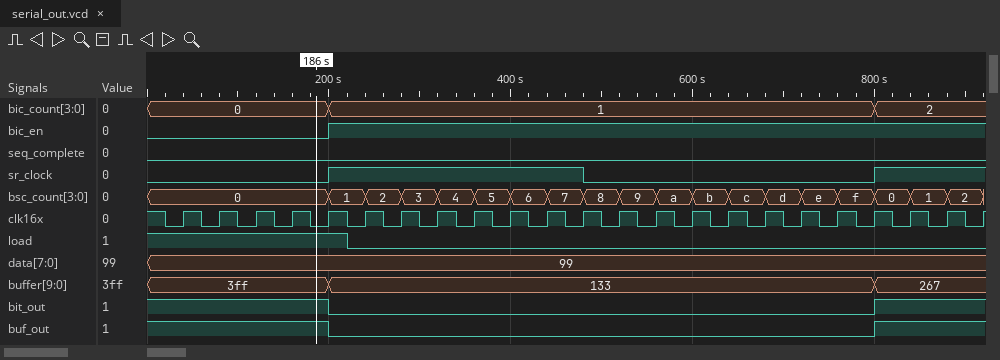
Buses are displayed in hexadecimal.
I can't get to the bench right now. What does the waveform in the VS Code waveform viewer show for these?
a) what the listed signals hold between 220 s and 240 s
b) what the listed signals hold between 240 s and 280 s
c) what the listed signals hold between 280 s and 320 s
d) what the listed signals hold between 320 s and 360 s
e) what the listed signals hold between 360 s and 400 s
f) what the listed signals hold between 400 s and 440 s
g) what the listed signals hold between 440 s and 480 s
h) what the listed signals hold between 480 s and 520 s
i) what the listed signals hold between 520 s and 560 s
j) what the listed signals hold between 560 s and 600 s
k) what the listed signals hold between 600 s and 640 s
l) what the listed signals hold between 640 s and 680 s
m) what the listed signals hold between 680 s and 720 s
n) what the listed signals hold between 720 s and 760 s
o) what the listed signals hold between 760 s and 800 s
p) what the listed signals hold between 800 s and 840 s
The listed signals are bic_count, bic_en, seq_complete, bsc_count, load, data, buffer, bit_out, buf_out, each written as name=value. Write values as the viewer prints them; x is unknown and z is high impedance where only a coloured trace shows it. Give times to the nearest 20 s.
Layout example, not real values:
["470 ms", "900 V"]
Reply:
["bic_count=1, bic_en=1, seq_complete=0, bsc_count=1, load=0, data=99, buffer=133, bit_out=0, buf_out=0", "bic_count=1, bic_en=1, seq_complete=0, bsc_count=2, load=0, data=99, buffer=133, bit_out=0, buf_out=0", "bic_count=1, bic_en=1, seq_complete=0, bsc_count=3, load=0, data=99, buffer=133, bit_out=0, buf_out=0", "bic_count=1, bic_en=1, seq_complete=0, bsc_count=4, load=0, data=99, buffer=133, bit_out=0, buf_out=0", "bic_count=1, bic_en=1, seq_complete=0, bsc_count=5, load=0, data=99, buffer=133, bit_out=0, buf_out=0", "bic_count=1, bic_en=1, seq_complete=0, bsc_count=6, load=0, data=99, buffer=133, bit_out=0, buf_out=0", "bic_count=1, bic_en=1, seq_complete=0, bsc_count=7, load=0, data=99, buffer=133, bit_out=0, buf_out=0", "bic_count=1, bic_en=1, seq_complete=0, bsc_count=8, load=0, data=99, buffer=133, bit_out=0, buf_out=0", "bic_count=1, bic_en=1, seq_complete=0, bsc_count=9, load=0, data=99, buffer=133, bit_out=0, buf_out=0", "bic_count=1, bic_en=1, seq_complete=0, bsc_count=a, load=0, data=99, buffer=133, bit_out=0, buf_out=0", "bic_count=1, bic_en=1, seq_complete=0, bsc_count=b, load=0, data=99, buffer=133, bit_out=0, buf_out=0", "bic_count=1, bic_en=1, seq_complete=0, bsc_count=c, load=0, data=99, buffer=133, bit_out=0, buf_out=0", "bic_count=1, bic_en=1, seq_complete=0, bsc_count=d, load=0, data=99, buffer=133, bit_out=0, buf_out=0", "bic_count=1, bic_en=1, seq_complete=0, bsc_count=e, load=0, data=99, buffer=133, bit_out=0, buf_out=0", "bic_count=1, bic_en=1, seq_complete=0, bsc_count=f, load=0, data=99, buffer=133, bit_out=0, buf_out=0", "bic_count=2, bic_en=1, seq_complete=0, bsc_count=0, load=0, data=99, buffer=267, bit_out=1, buf_out=1"]
